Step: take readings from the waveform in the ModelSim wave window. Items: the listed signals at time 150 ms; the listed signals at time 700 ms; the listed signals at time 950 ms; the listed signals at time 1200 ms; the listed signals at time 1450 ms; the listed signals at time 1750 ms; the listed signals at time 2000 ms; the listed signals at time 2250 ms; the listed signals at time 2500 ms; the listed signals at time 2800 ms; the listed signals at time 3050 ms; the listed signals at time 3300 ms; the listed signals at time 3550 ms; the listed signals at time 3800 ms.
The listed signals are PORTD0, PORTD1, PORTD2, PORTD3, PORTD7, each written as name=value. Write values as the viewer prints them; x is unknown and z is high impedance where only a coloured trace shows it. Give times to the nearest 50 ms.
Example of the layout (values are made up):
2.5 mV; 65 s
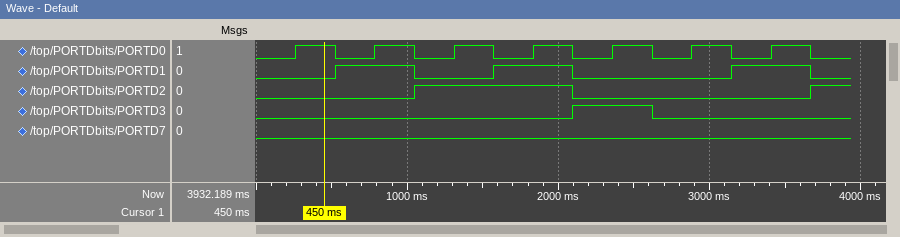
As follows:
PORTD0=0, PORTD1=0, PORTD2=0, PORTD3=0, PORTD7=0; PORTD0=0, PORTD1=1, PORTD2=0, PORTD3=0, PORTD7=0; PORTD0=1, PORTD1=1, PORTD2=0, PORTD3=0, PORTD7=0; PORTD0=0, PORTD1=0, PORTD2=1, PORTD3=0, PORTD7=0; PORTD0=1, PORTD1=0, PORTD2=1, PORTD3=0, PORTD7=0; PORTD0=0, PORTD1=1, PORTD2=1, PORTD3=0, PORTD7=0; PORTD0=1, PORTD1=1, PORTD2=1, PORTD3=0, PORTD7=0; PORTD0=0, PORTD1=0, PORTD2=0, PORTD3=1, PORTD7=0; PORTD0=1, PORTD1=0, PORTD2=0, PORTD3=1, PORTD7=0; PORTD0=0, PORTD1=0, PORTD2=0, PORTD3=0, PORTD7=0; PORTD0=1, PORTD1=0, PORTD2=0, PORTD3=0, PORTD7=0; PORTD0=0, PORTD1=1, PORTD2=0, PORTD3=0, PORTD7=0; PORTD0=1, PORTD1=1, PORTD2=0, PORTD3=0, PORTD7=0; PORTD0=0, PORTD1=0, PORTD2=1, PORTD3=0, PORTD7=0
